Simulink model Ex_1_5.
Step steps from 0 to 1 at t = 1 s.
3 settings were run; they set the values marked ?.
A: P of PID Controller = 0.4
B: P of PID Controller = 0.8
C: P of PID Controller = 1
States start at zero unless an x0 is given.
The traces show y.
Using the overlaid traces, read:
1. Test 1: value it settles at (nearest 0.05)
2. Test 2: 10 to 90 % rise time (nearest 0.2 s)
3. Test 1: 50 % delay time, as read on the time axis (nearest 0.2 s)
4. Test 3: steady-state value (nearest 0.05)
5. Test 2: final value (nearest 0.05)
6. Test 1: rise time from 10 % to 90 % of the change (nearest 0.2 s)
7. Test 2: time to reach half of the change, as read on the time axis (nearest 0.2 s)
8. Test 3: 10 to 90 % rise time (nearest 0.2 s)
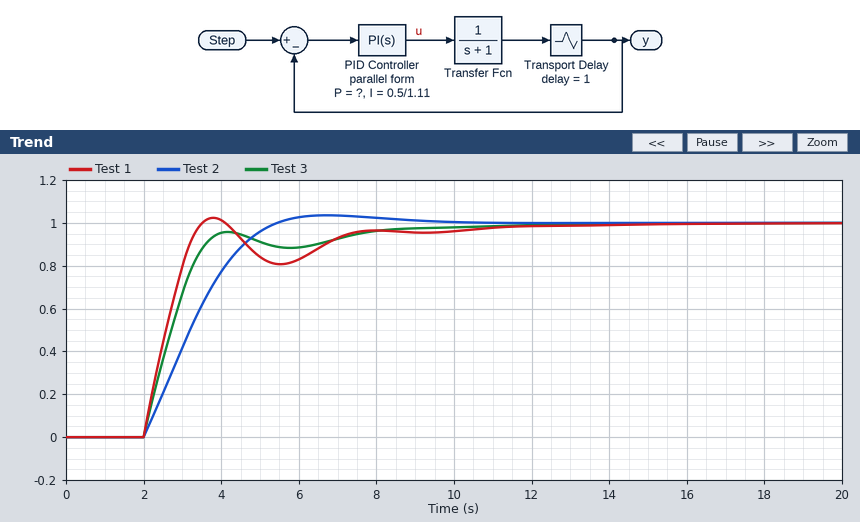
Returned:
1.00
2.4 s
2.6 s
1.00
1.00
1.0 s
3.2 s
1.4 s
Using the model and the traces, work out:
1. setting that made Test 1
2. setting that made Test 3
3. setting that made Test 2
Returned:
C
B
A
